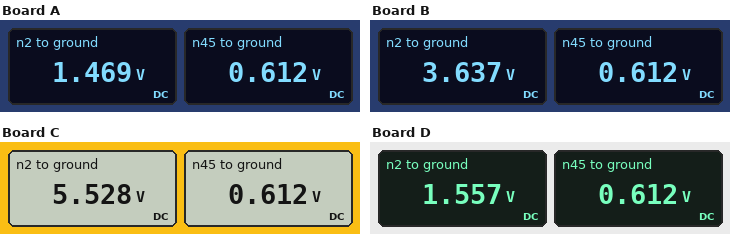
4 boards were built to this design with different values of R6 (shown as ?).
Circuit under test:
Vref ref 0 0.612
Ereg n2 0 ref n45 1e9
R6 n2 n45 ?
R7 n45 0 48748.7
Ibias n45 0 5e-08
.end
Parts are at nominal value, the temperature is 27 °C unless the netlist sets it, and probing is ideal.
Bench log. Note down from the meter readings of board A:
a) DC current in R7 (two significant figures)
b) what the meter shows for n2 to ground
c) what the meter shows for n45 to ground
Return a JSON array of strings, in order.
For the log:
["13 µA", "1.469 V", "0.612 V"]
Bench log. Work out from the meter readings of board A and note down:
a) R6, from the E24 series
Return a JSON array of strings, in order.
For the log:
["68 kΩ"]
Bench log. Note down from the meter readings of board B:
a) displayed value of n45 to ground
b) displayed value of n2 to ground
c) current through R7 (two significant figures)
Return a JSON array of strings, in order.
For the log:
["0.612 V", "3.637 V", "13 µA"]
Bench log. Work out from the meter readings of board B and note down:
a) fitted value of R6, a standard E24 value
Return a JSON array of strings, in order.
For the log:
["240 kΩ"]
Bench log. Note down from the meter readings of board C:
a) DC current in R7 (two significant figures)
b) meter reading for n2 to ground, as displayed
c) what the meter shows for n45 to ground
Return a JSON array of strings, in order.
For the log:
["13 µA", "5.528 V", "0.612 V"]
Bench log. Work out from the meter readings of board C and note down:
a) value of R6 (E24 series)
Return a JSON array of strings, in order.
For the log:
["390 kΩ"]
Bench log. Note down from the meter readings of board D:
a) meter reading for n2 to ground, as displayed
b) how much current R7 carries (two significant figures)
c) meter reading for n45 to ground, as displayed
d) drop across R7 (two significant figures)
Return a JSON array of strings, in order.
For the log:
["1.557 V", "13 µA", "0.612 V", "610 mV"]
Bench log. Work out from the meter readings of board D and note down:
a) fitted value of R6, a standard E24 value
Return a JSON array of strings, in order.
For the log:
["75 kΩ"]
